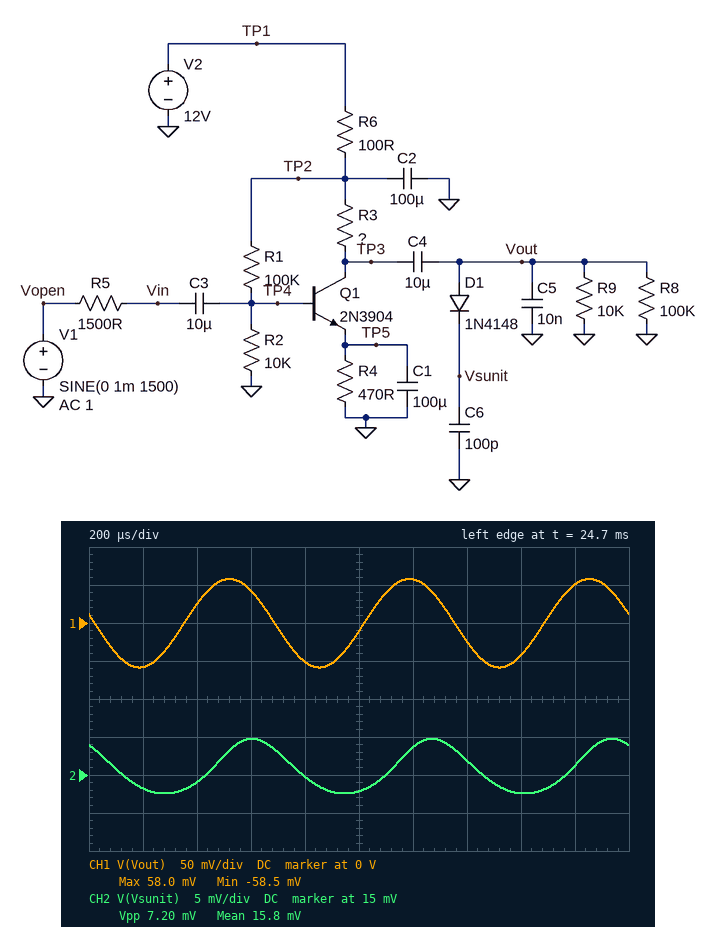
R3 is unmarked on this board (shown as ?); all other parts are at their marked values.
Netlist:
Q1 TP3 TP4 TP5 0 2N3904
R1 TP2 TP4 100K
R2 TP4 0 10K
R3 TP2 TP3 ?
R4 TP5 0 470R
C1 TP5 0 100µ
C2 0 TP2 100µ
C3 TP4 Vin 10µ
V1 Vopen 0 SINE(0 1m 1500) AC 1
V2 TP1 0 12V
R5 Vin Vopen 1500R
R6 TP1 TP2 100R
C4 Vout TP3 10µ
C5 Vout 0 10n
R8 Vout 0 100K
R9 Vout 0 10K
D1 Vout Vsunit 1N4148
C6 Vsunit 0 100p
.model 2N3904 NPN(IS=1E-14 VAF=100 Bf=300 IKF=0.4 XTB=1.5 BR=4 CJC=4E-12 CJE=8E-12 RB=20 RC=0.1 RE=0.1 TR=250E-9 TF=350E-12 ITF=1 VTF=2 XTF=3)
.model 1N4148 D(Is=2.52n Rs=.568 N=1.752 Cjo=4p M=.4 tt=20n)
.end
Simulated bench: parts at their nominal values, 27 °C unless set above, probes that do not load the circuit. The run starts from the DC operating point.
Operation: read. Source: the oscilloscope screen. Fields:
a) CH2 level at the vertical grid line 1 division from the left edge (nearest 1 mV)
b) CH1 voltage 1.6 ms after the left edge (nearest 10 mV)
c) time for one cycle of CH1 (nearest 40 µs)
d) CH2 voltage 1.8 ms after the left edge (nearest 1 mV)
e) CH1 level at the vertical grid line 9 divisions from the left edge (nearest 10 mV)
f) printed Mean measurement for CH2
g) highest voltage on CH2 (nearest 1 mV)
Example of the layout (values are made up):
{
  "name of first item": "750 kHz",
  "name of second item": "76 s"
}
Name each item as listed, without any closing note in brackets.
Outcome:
{
  "CH2 level at the vertical grid line 1 division from the left edge": "13 mV",
  "CH1 voltage 1.6 ms after the left edge": "-40 mV",
  "time for one cycle of CH1": "680 µs",
  "CH2 voltage 1.8 ms after the left edge": "16 mV",
  "CH1 level at the vertical grid line 9 divisions from the left edge": "50 mV",
  "printed Mean measurement for CH2": "15.8 mV",
  "highest voltage on CH2": "20 mV"
}
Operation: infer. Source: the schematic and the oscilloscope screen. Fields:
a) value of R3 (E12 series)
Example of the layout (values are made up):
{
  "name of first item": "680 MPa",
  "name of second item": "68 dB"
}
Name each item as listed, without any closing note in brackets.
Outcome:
{
  "value of R3": "3.3 kΩ"
}
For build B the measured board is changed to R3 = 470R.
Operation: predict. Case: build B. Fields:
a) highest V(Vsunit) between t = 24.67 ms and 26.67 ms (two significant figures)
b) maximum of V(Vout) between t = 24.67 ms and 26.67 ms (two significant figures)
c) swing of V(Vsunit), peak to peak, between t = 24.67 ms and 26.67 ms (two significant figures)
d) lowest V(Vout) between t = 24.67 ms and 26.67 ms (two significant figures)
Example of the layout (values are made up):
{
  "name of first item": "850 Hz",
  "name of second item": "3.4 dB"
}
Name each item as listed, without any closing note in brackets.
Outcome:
{
  "highest V(Vsunit) between t = 24.67 ms and 26.67 ms": "1.4 mV",
  "maximum of V(Vout) between t = 24.67 ms and 26.67 ms": "11 mV",
  "swing of V(Vsunit), peak to peak, between t = 24.67 ms and 26.67 ms": "1.5 mV",
  "lowest V(Vout) between t = 24.67 ms and 26.67 ms": "-11 mV"
}
